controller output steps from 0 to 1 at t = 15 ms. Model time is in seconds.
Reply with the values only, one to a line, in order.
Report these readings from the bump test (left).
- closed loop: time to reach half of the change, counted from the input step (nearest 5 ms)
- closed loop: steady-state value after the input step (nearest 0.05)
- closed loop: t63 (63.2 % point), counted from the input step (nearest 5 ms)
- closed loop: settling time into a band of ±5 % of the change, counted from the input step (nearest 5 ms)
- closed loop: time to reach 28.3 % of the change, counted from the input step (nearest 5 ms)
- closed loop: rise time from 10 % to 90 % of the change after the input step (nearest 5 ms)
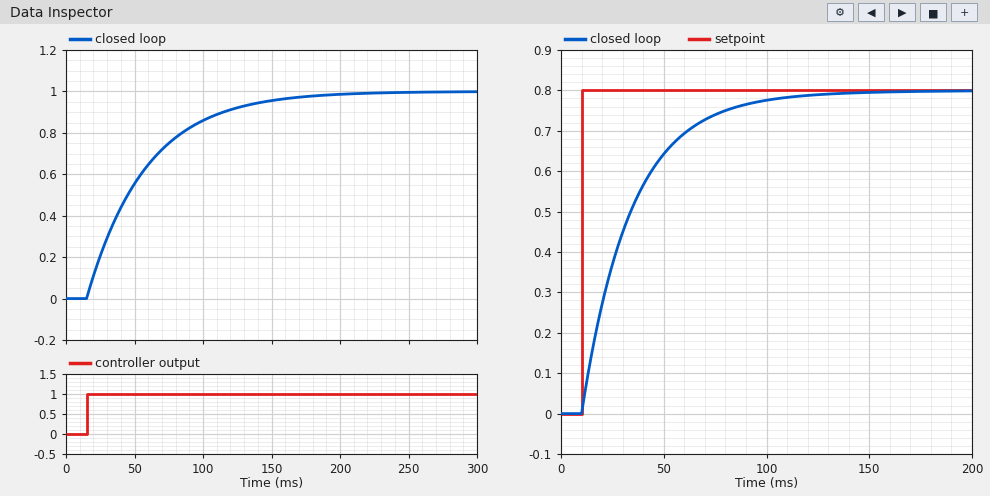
30 ms
1.00
45 ms
130 ms
15 ms
95 ms
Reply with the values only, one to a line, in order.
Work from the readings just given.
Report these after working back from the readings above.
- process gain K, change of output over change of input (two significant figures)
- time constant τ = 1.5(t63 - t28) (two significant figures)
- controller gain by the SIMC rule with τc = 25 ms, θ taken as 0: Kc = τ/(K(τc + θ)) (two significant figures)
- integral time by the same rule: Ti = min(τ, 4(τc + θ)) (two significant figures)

1.0
45 ms
1.8
45 ms
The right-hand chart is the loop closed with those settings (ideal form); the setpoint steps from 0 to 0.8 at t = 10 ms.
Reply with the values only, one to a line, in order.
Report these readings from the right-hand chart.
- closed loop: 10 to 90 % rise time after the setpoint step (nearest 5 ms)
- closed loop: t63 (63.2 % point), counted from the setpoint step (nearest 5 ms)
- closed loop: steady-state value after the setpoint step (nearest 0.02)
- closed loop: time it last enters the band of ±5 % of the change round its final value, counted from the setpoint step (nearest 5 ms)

55 ms
25 ms
0.80
75 ms
